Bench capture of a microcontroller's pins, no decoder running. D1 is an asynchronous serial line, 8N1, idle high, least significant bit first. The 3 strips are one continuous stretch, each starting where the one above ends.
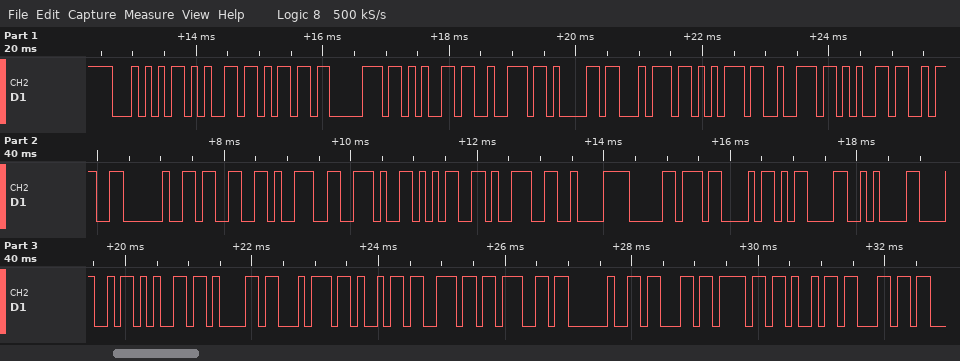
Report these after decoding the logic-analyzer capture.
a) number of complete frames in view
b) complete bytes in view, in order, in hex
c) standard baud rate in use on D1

35
54 65 6D 70 65 72 61 74 75 72 65 3A 20 33 39 2E 35 39 C2 B0 43 0D 0A 48 65 61 74 69 6E 67 20 63 6F 69 6C
9600 baud
